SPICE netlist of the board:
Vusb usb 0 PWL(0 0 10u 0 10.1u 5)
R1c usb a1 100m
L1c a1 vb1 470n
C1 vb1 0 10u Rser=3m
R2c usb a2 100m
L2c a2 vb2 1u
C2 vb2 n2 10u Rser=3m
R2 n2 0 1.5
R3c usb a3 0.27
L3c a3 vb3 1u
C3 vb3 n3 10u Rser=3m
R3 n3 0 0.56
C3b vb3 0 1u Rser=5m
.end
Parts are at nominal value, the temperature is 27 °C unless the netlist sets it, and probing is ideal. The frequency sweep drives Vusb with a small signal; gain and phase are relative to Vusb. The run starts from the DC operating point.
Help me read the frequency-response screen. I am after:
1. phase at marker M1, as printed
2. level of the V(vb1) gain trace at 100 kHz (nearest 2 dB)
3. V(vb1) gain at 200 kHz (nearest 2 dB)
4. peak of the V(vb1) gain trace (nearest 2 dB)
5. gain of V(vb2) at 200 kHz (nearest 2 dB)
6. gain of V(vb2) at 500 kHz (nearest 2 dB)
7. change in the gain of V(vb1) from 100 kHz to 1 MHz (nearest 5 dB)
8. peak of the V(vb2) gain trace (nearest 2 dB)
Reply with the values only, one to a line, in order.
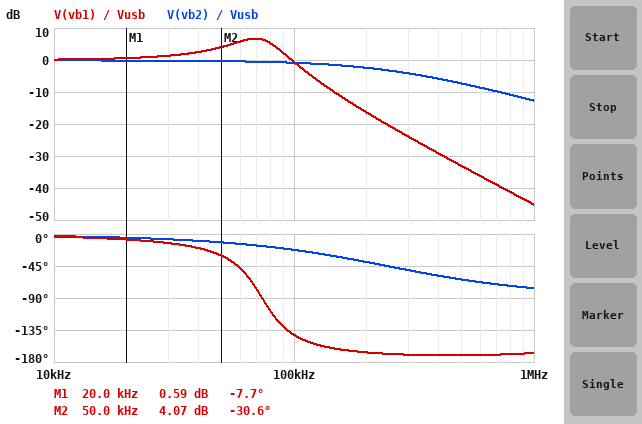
-7.7 deg
0 dB
-16 dB
6 dB
-2 dB
-8 dB
-45 dB
0 dB
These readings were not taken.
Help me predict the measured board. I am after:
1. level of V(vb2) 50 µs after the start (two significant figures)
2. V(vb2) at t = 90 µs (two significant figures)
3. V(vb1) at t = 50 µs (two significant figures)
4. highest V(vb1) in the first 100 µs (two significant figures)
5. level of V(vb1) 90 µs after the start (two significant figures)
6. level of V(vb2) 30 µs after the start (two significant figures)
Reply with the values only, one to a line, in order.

5.0 V
5.0 V
5.0 V
7.3 V
5.0 V
5.0 V
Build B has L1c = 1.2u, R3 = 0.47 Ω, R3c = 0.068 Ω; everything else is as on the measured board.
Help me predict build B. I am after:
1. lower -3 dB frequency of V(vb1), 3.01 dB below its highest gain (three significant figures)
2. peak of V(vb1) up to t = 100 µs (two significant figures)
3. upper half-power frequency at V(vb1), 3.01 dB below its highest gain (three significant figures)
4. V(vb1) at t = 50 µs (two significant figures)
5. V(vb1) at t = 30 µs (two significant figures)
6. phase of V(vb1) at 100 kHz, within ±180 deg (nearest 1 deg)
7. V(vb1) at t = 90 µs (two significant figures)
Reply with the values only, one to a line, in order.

37.4 kHz
8.1 V
51.4 kHz
4.8 V
3.4 V
-169 deg
5.1 V
